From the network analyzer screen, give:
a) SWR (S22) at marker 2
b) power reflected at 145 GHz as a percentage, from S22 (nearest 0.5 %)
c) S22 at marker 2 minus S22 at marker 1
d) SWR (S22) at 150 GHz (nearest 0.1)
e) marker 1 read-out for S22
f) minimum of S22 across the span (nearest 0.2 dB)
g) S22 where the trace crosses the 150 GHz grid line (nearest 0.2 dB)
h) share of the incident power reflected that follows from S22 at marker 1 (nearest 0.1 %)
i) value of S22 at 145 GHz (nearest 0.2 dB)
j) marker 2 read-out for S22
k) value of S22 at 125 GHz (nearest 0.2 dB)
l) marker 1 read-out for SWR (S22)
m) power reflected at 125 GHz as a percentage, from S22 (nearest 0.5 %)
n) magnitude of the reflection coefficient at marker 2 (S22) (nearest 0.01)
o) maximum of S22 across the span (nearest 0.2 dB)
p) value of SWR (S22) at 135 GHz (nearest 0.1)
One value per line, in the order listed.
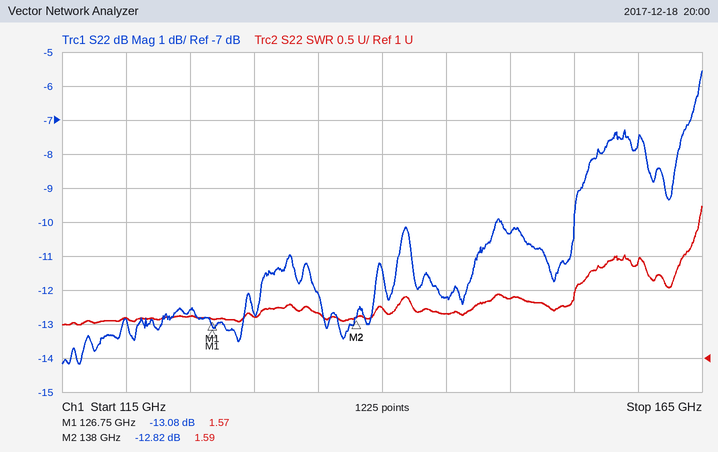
1.59
6.0 %
0.26 dB
1.9
-13.08 dB
-14.2 dB
-10.4 dB
4.9 %
-12.2 dB
-12.82 dB
-12.6 dB
1.57
5.5 %
0.23
-5.6 dB
1.7
